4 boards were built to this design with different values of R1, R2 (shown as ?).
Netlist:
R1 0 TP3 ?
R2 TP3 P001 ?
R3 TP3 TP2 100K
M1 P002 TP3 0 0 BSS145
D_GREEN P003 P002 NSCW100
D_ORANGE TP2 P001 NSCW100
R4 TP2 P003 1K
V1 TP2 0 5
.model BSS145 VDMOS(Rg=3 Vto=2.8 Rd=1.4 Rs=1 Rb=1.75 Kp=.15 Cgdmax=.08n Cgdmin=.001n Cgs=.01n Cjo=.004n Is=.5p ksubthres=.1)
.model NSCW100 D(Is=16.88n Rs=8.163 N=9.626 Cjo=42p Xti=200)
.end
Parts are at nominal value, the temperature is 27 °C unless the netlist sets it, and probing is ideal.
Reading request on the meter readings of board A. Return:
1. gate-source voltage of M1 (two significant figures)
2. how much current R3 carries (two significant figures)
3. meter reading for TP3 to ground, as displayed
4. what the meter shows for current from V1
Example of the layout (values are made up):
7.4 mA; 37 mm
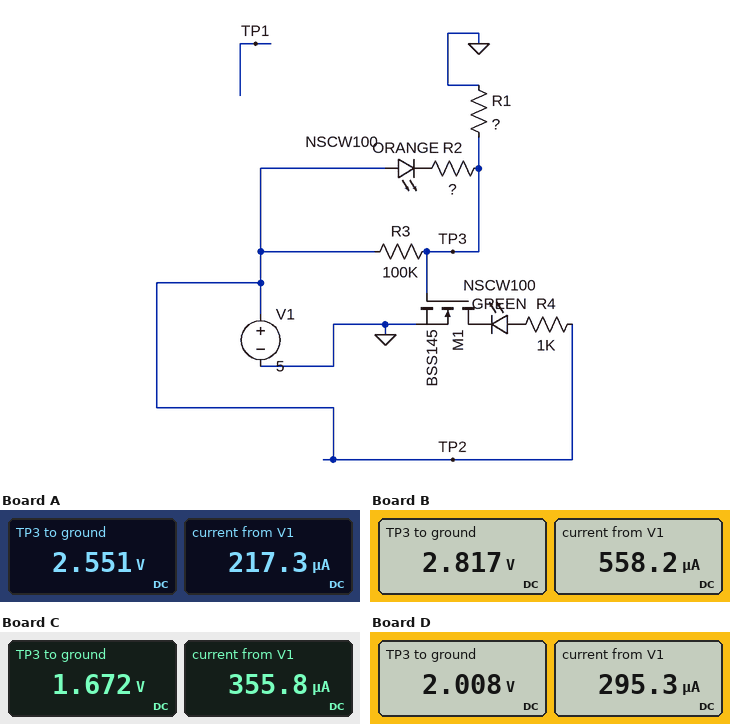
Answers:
2.6 V; 24 µA; 2.551 V; 217.3 µA
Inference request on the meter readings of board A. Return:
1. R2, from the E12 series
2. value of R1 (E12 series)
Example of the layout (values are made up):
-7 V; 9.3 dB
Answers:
680 Ω; 12 kΩ
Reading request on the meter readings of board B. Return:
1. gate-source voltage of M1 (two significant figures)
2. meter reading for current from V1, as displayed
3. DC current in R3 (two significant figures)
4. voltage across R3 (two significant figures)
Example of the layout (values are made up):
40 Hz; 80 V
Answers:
2.8 V; 558.2 µA; 22 µA; 2.2 V
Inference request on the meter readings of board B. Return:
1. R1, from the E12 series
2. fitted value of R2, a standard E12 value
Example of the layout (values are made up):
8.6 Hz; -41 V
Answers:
27 kΩ; 820 Ω
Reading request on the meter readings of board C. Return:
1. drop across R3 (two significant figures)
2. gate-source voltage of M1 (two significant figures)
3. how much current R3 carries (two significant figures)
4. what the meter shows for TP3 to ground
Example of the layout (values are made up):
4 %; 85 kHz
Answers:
3.3 V; 1.7 V; 33 µA; 1.672 V
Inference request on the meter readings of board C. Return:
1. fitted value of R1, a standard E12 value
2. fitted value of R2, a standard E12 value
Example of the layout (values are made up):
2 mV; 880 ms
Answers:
4.7 kΩ; 2.7 kΩ
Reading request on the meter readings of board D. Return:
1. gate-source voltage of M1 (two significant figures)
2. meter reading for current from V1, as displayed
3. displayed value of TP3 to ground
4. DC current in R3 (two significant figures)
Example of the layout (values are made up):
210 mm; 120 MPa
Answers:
2.0 V; 295.3 µA; 2.008 V; 30 µA
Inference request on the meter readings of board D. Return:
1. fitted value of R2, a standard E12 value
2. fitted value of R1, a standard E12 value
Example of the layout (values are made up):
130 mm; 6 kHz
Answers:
2.2 kΩ; 6.8 kΩ
